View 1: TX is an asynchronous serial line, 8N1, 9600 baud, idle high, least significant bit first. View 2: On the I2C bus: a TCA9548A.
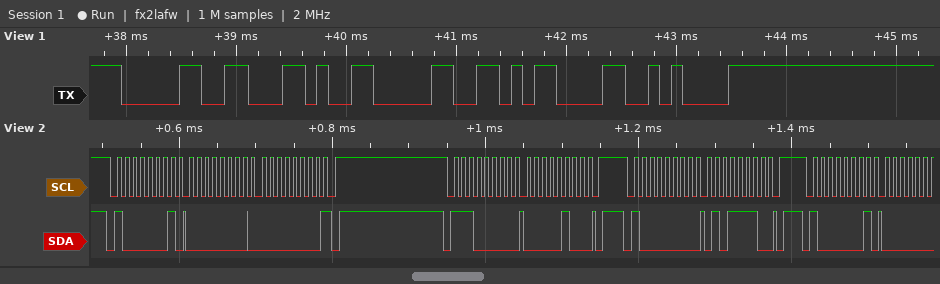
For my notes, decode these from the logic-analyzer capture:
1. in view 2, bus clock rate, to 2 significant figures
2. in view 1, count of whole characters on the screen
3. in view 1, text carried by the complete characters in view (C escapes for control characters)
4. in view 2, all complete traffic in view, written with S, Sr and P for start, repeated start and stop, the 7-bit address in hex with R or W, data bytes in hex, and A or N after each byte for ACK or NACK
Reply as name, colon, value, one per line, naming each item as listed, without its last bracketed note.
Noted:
in view 2, bus clock rate, to 2 significant figures: 100 kHz
in view 1, count of whole characters on the screen: 5
in view 1, text carried by the complete characters in view: "0,0\r\n"
in view 2, all complete traffic in view, written with S, Sr and P for start, repeated start and stop, the 7-bit address in hex with R or W, data bytes in hex, and A or N after each byte for ACK or NACK: S 40R A 00 A 00 N P S 70W A 04 A P S 40W A 5E A P S 40R A
